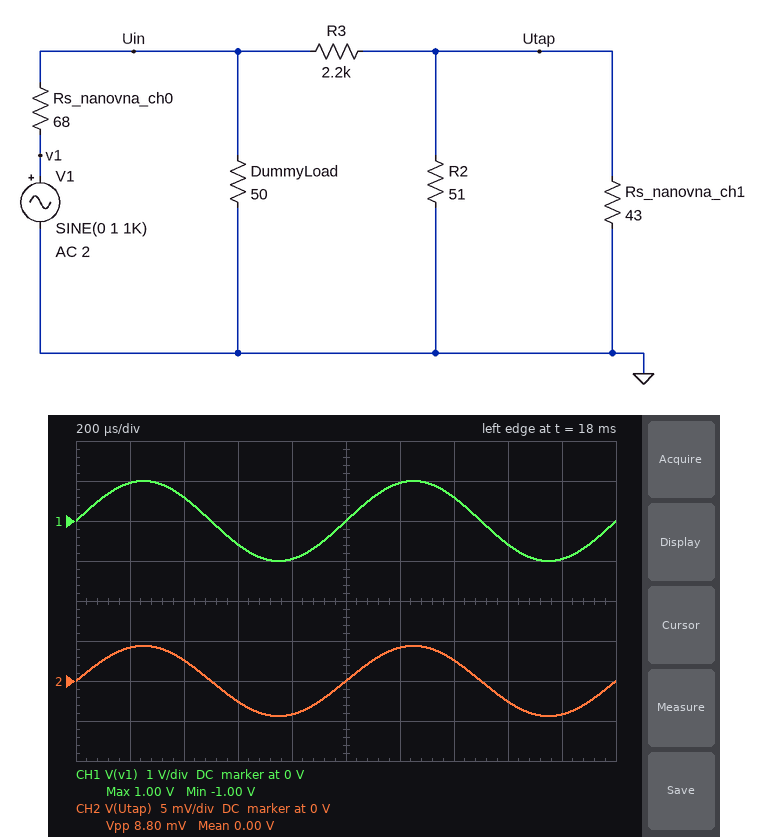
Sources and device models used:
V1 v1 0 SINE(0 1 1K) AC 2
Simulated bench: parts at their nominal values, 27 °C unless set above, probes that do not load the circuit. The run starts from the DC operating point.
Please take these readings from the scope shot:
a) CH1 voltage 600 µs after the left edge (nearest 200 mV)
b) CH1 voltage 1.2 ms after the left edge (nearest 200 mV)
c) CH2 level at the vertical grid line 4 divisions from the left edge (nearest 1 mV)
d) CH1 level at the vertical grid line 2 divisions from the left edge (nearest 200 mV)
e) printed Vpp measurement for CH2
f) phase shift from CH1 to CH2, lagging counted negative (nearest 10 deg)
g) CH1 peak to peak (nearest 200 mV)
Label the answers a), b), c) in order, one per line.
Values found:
a) -600 mV
b) 1.0 V
c) -4 mV
d) 600 mV
e) 8.80 mV
f) 0 deg
g) 2.0 V
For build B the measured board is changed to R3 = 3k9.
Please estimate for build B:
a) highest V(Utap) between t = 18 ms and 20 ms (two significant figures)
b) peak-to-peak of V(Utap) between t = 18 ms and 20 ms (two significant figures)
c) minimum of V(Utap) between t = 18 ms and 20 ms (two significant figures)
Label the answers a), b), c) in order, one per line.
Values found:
a) 2.5 mV
b) 5.0 mV
c) -2.5 mV
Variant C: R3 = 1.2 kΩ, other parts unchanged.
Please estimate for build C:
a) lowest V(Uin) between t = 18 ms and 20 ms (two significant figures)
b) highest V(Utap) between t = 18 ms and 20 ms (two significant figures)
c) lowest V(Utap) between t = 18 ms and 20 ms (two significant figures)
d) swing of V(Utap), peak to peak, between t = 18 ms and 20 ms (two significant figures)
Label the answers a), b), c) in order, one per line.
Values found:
a) -410 mV
b) 7.9 mV
c) -7.9 mV
d) 16 mV
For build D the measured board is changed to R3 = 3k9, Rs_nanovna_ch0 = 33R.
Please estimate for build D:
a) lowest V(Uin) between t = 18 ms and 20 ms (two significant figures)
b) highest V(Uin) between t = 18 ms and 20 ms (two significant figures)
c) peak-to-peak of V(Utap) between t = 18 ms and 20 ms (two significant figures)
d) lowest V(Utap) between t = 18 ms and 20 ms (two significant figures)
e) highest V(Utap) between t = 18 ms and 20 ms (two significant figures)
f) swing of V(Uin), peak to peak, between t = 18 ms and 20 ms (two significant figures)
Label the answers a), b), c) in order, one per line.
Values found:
a) -600 mV
b) 600 mV
c) 7.1 mV
d) -3.6 mV
e) 3.6 mV
f) 1.2 V
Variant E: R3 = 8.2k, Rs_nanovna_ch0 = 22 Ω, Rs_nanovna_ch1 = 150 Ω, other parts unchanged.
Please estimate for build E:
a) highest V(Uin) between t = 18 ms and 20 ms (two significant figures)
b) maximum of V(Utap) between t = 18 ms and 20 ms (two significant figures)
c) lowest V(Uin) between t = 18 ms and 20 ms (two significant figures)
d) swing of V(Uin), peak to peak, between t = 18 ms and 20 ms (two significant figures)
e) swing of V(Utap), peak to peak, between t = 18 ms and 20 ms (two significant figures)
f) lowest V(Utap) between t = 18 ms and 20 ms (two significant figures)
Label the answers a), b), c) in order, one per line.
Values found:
a) 690 mV
b) 3.2 mV
c) -690 mV
d) 1.4 V
e) 6.4 mV
f) -3.2 mV
